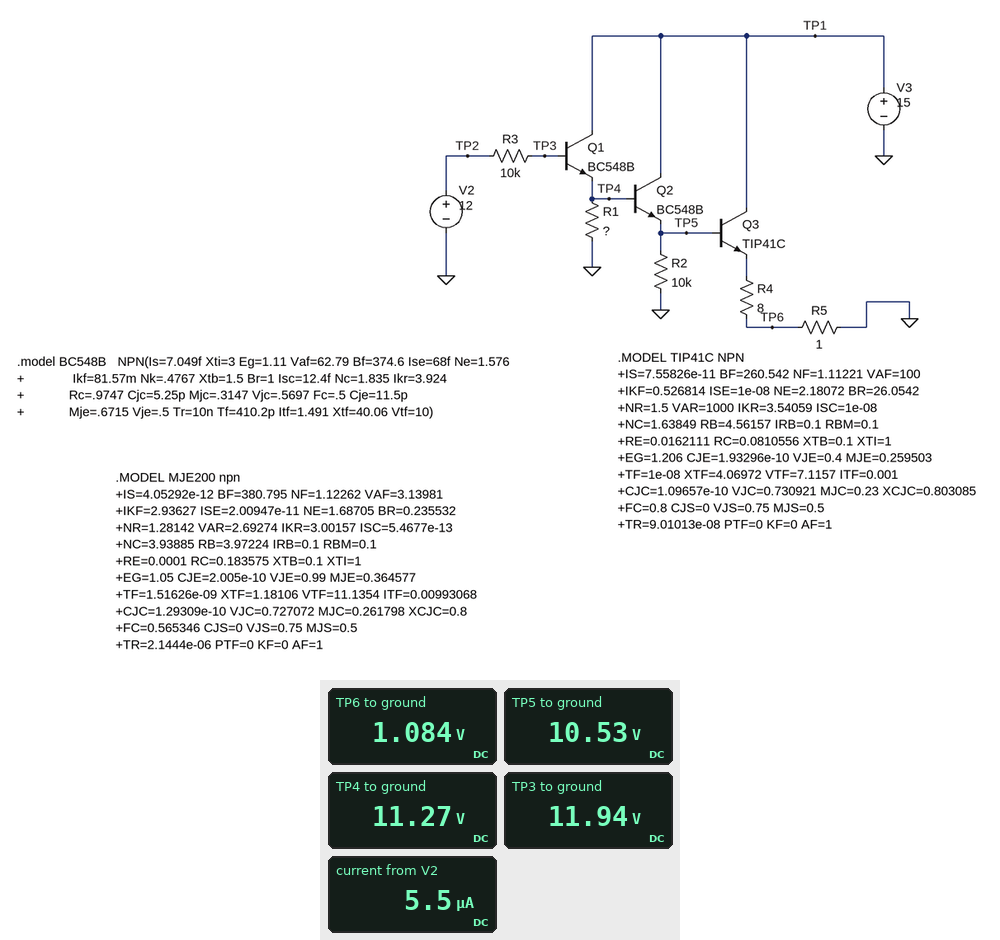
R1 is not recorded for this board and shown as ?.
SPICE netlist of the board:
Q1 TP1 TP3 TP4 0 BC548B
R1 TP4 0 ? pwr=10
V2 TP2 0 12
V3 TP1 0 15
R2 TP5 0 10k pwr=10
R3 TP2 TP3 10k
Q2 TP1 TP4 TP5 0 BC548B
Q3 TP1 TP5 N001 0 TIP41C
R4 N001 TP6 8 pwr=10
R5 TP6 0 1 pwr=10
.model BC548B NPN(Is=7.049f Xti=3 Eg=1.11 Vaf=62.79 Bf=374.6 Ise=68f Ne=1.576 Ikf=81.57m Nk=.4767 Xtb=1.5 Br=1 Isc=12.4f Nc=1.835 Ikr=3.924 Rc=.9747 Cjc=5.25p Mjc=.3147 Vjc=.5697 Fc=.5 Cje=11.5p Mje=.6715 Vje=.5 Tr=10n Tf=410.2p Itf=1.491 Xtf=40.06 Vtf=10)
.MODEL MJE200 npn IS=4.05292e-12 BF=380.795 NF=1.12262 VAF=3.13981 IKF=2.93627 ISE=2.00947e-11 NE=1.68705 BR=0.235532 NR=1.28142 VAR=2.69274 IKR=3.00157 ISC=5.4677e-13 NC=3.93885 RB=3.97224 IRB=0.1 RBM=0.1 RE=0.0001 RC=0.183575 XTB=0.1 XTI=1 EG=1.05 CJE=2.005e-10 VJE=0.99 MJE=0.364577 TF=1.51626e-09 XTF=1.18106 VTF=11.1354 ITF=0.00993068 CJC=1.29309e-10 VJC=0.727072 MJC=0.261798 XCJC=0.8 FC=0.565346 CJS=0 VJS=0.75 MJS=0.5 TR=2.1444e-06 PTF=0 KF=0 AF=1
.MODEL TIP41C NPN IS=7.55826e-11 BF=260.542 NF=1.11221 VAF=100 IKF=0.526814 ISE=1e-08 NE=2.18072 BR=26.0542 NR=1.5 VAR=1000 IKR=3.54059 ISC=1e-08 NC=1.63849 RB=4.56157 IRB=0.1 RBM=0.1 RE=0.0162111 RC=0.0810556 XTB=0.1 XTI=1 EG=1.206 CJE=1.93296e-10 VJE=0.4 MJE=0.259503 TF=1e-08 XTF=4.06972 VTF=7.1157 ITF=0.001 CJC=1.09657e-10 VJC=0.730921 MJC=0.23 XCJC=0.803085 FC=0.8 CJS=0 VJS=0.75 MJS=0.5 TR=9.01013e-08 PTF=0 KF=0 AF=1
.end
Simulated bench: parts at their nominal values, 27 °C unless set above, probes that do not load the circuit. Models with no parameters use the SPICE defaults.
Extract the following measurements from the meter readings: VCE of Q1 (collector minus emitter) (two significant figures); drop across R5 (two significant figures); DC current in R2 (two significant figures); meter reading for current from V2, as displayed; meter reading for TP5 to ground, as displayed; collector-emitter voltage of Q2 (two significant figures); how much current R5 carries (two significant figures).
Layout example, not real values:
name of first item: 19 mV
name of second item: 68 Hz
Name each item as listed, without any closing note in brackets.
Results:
VCE of Q1 (collector minus emitter): 3.7 V
drop across R5: 1.1 V
DC current in R2: 1.1 mA
meter reading for current from V2, as displayed: 5.5 µA
meter reading for TP5 to ground, as displayed: 10.53 V
collector-emitter voltage of Q2: 4.5 V
how much current R5 carries: 1.1 A
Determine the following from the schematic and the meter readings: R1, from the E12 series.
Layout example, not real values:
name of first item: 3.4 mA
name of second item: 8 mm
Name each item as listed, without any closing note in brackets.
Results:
R1, from the E12 series: 6.8 kΩ
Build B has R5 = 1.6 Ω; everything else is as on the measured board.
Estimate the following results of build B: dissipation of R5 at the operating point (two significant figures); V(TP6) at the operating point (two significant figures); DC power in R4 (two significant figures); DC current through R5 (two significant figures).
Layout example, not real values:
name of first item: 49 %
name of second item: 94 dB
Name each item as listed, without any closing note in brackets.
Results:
dissipation of R5 at the operating point: 1.7 W
V(TP6) at the operating point: 1.6 V
DC power in R4: 8.3 W
DC current through R5: 1.0 A
